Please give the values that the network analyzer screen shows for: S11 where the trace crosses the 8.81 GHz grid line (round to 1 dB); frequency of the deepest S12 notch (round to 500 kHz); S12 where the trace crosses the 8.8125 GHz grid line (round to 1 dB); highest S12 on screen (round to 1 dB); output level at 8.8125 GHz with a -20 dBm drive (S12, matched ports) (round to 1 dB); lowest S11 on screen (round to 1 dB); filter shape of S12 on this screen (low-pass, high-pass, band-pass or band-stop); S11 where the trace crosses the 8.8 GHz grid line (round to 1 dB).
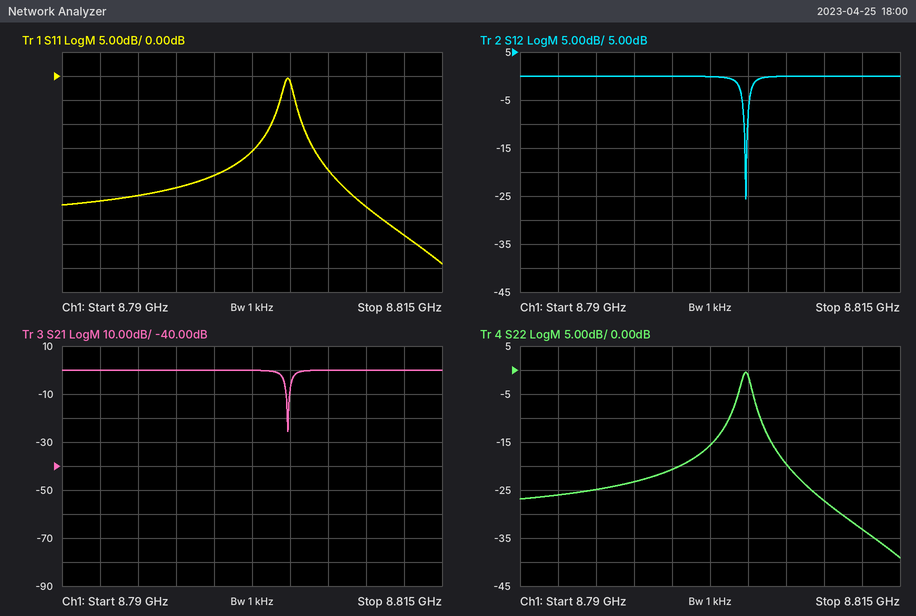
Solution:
-27 dB
8.8050 GHz
0 dB
0 dB
-20 dBm
-39 dB
band-stop
-21 dB
